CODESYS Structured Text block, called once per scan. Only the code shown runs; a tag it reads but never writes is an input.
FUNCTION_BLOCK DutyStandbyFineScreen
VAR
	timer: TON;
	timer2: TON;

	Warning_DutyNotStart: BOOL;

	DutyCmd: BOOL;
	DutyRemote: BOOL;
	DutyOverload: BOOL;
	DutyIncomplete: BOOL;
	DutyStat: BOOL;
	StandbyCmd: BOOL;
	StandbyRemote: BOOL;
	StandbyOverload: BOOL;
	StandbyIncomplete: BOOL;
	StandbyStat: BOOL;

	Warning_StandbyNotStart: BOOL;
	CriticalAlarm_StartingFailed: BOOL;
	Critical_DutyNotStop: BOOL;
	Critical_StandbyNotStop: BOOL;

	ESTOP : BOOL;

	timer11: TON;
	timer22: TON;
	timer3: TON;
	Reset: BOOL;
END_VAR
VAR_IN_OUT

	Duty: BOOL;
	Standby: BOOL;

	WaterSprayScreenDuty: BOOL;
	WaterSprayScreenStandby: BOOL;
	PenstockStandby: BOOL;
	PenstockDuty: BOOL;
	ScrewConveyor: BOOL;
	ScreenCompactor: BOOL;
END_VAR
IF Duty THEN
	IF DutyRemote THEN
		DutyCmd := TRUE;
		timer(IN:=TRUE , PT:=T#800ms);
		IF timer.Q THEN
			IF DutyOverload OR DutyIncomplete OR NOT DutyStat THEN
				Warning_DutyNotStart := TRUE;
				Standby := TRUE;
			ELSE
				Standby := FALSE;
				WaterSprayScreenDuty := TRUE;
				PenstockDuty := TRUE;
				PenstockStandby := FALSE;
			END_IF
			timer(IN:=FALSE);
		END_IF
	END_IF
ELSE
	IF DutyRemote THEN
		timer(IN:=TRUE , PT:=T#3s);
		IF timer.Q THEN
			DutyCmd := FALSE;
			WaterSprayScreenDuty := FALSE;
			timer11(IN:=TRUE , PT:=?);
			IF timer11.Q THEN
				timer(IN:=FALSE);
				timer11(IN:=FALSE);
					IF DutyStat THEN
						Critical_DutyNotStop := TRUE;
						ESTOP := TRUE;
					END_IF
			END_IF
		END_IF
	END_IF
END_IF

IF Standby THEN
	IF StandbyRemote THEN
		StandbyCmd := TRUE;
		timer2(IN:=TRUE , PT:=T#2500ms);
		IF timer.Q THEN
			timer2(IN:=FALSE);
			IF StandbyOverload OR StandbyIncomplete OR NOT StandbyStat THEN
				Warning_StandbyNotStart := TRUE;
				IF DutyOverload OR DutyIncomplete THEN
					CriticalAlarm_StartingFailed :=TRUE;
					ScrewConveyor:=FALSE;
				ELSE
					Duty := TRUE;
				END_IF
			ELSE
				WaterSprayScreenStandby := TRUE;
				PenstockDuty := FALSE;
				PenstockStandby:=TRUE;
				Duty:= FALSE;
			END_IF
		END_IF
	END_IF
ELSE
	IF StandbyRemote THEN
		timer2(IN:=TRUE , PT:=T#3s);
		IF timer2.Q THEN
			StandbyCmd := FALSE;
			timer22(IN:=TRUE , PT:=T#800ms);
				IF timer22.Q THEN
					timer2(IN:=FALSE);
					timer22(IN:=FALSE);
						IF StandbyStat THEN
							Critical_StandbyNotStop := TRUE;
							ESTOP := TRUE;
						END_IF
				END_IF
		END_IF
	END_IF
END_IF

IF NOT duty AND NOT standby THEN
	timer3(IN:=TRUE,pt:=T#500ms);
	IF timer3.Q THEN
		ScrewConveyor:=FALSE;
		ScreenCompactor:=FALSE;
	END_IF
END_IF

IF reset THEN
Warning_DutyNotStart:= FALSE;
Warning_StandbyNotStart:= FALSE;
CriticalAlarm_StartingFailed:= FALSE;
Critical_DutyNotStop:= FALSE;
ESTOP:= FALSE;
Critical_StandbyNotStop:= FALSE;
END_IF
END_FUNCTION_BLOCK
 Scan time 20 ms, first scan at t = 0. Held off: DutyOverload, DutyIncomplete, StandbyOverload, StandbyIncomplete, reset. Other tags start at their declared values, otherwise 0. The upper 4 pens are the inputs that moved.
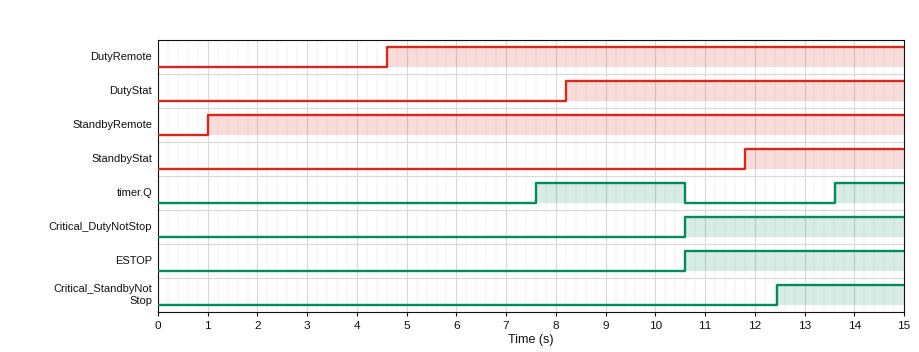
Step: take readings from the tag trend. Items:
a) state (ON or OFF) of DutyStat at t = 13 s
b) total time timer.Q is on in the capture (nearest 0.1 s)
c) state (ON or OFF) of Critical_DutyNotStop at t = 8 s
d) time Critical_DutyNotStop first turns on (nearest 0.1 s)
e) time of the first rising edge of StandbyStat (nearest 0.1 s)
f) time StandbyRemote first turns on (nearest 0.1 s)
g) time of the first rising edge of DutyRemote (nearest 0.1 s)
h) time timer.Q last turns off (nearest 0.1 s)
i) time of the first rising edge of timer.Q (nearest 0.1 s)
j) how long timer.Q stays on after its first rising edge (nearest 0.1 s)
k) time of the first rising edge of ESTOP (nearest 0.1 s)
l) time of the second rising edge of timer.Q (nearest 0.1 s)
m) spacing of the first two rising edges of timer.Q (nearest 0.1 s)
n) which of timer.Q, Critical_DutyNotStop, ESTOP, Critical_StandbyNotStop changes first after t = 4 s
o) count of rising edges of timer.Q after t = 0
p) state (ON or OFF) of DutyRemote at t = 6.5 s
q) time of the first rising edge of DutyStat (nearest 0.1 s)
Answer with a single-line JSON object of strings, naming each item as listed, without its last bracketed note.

{"state (ON or OFF) of DutyStat at t = 13 s": "ON", "total time timer.Q is on in the capture": "4.4 s", "state (ON or OFF) of Critical_DutyNotStop at t = 8 s": "OFF", "time Critical_DutyNotStop first turns on": "10.6 s", "time of the first rising edge of StandbyStat": "11.8 s", "time StandbyRemote first turns on": "1.0 s", "time of the first rising edge of DutyRemote": "4.6 s", "time timer.Q last turns off": "10.6 s", "time of the first rising edge of timer.Q": "7.6 s", "how long timer.Q stays on after its first rising edge": "3.0 s", "time of the first rising edge of ESTOP": "10.6 s", "time of the second rising edge of timer.Q": "13.6 s", "spacing of the first two rising edges of timer.Q": "6.0 s", "which of timer.Q, Critical_DutyNotStop, ESTOP, Critical_StandbyNotStop changes first after t = 4 s": "timer.Q", "count of rising edges of timer.Q after t = 0": "2", "state (ON or OFF) of DutyRemote at t = 6.5 s": "ON", "time of the first rising edge of DutyStat": "8.2 s"}
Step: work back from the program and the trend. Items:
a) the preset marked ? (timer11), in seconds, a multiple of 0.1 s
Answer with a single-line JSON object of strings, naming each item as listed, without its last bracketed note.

{"the preset marked ? (timer11), in seconds, a multiple of 0.1 s": "3.0 s"}
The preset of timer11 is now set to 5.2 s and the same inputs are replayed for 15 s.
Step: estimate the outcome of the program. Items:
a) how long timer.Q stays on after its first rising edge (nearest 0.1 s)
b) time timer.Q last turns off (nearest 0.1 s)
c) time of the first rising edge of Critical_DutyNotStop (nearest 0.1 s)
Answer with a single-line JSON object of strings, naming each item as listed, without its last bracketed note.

{"how long timer.Q stays on after its first rising edge": "5.2 s", "time timer.Q last turns off": "12.8 s", "time of the first rising edge of Critical_DutyNotStop": "12.8 s"}
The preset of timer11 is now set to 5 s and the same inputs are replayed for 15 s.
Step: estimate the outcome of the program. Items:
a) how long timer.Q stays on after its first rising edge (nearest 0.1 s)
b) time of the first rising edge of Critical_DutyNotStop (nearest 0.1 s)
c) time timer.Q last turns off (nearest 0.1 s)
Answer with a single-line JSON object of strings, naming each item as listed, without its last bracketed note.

{"how long timer.Q stays on after its first rising edge": "5.0 s", "time of the first rising edge of Critical_DutyNotStop": "12.6 s", "time timer.Q last turns off": "12.6 s"}
